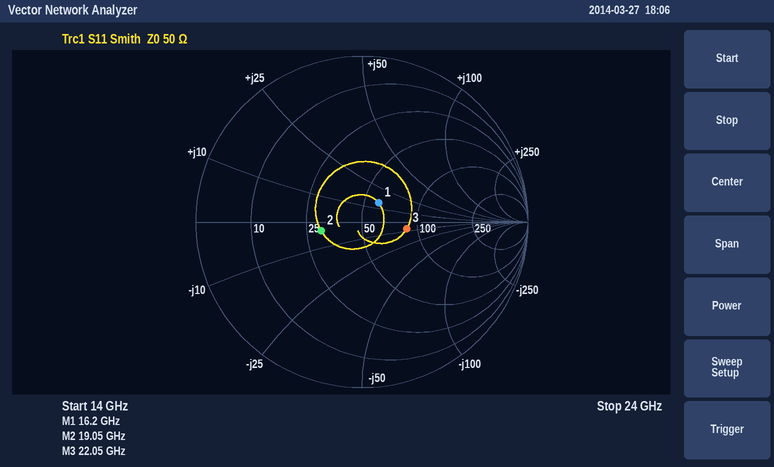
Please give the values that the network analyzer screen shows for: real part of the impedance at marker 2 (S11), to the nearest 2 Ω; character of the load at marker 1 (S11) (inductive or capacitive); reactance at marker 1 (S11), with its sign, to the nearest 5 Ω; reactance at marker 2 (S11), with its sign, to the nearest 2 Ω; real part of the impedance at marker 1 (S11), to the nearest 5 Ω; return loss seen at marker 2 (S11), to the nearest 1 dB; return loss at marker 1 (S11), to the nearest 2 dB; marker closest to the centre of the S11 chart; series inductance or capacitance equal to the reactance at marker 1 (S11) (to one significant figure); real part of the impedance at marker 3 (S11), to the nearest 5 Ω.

30 Ω
inductive
+15 Ω
-4 Ω
60 Ω
12 dB
16 dB
marker 1
100 pH
85 Ω
